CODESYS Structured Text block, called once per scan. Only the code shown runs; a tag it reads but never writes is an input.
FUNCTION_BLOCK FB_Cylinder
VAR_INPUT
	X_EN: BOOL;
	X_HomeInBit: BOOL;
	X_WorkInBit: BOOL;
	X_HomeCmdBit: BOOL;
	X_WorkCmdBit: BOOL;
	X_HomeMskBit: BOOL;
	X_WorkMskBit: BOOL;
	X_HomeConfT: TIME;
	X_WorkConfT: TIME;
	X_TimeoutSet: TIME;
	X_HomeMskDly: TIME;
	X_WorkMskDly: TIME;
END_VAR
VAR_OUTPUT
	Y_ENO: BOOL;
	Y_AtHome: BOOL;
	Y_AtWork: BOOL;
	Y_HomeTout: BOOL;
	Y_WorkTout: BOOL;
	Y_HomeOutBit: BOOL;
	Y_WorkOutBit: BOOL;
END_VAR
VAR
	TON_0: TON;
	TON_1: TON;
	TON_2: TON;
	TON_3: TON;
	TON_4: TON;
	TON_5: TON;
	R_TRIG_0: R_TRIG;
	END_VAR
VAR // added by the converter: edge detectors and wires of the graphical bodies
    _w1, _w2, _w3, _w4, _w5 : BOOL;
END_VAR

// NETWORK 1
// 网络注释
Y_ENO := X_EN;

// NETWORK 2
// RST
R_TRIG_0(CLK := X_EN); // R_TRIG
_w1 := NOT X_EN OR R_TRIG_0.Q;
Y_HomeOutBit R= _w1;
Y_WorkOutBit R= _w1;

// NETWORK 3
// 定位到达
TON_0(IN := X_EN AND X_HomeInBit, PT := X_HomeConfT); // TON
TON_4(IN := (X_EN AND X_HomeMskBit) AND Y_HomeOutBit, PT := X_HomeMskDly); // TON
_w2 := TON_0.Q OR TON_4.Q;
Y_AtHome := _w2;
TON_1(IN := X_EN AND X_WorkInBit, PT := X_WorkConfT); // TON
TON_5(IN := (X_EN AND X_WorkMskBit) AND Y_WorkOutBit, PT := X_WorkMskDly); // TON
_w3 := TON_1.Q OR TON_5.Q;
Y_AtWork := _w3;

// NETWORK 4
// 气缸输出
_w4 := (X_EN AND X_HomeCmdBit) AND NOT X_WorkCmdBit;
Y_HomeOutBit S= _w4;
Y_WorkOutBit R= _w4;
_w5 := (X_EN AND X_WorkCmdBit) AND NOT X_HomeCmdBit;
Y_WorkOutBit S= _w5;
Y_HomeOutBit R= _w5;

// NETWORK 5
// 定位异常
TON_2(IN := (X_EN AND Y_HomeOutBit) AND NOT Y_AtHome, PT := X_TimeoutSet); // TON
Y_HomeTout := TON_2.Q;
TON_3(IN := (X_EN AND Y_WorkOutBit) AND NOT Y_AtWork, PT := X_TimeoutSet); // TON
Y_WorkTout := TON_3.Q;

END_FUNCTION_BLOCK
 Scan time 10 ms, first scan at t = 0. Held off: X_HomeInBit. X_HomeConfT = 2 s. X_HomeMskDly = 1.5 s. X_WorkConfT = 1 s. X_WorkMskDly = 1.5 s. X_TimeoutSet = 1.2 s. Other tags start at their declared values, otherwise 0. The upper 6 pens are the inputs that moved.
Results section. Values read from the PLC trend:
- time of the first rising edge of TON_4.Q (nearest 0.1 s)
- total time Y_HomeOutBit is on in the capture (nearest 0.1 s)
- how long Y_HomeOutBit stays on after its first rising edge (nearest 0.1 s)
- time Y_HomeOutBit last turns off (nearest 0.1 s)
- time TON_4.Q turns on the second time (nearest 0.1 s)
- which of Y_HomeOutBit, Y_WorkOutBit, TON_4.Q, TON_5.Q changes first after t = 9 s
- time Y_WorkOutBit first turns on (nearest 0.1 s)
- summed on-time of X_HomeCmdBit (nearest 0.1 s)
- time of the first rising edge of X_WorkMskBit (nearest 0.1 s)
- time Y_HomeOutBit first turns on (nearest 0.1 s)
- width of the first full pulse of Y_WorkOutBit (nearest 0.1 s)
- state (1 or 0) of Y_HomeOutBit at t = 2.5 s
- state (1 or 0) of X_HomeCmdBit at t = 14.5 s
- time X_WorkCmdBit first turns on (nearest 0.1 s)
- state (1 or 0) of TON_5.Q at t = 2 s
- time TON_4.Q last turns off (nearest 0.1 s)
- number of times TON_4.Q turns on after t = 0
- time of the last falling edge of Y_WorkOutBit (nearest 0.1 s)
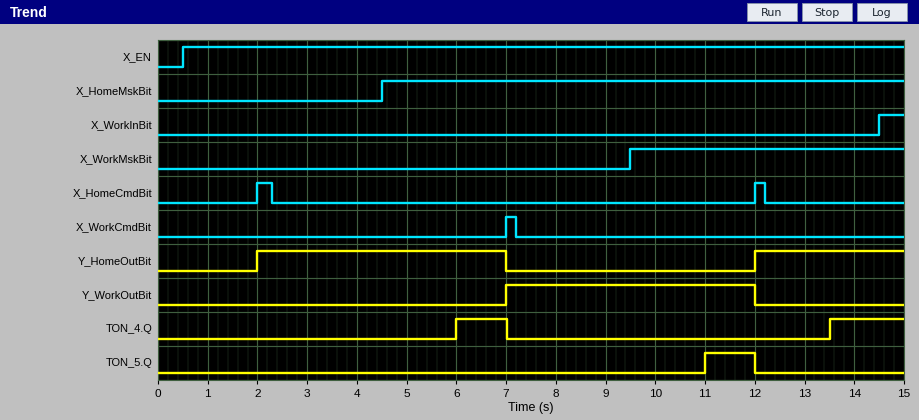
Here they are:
6.0 s
8.0 s
5.0 s
7.0 s
13.5 s
TON_5.Q
7.0 s
0.5 s
9.5 s
2.0 s
5.0 s
1
0
7.0 s
0
7.0 s
2
12.0 s
